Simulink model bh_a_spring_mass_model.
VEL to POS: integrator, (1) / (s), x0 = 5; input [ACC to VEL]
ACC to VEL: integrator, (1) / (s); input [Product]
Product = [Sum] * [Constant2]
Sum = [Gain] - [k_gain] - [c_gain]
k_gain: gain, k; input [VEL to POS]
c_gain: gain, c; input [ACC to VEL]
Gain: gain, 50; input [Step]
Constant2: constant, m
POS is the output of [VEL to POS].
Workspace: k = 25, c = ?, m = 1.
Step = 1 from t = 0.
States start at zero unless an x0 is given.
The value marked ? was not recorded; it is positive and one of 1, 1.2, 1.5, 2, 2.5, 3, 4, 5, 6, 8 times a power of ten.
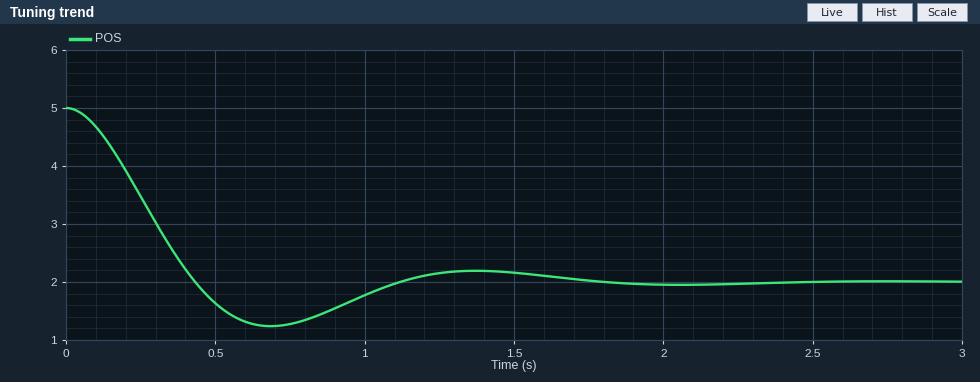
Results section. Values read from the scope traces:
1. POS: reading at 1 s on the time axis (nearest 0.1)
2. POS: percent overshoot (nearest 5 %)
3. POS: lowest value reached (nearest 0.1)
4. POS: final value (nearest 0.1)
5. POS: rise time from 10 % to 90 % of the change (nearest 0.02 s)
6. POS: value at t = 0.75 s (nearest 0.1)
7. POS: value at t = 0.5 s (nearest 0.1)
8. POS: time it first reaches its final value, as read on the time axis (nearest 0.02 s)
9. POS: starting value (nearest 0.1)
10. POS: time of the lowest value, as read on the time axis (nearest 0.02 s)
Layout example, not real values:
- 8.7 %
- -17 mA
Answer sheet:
- 1.8
- 25 %
- 1.2
- 2.0
- 0.30 s
- 1.3
- 1.6
- 0.44 s
- 5.0
- 0.68 s
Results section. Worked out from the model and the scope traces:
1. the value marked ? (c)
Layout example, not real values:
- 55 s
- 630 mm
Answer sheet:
- 4
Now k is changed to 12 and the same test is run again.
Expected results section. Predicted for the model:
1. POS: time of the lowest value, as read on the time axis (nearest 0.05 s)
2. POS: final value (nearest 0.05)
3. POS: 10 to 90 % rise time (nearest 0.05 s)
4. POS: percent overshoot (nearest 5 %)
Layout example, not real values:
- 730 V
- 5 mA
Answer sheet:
- 1.10 s
- 4.15
- 0.50 s
- 10 %
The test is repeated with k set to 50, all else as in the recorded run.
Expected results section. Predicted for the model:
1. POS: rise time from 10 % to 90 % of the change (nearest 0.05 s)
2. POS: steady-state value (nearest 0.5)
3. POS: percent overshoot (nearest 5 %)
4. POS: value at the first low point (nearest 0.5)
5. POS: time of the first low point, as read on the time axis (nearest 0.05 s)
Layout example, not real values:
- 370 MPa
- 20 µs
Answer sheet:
- 0.20 s
- 1.0
- 40 %
- -0.5
- 0.45 s
